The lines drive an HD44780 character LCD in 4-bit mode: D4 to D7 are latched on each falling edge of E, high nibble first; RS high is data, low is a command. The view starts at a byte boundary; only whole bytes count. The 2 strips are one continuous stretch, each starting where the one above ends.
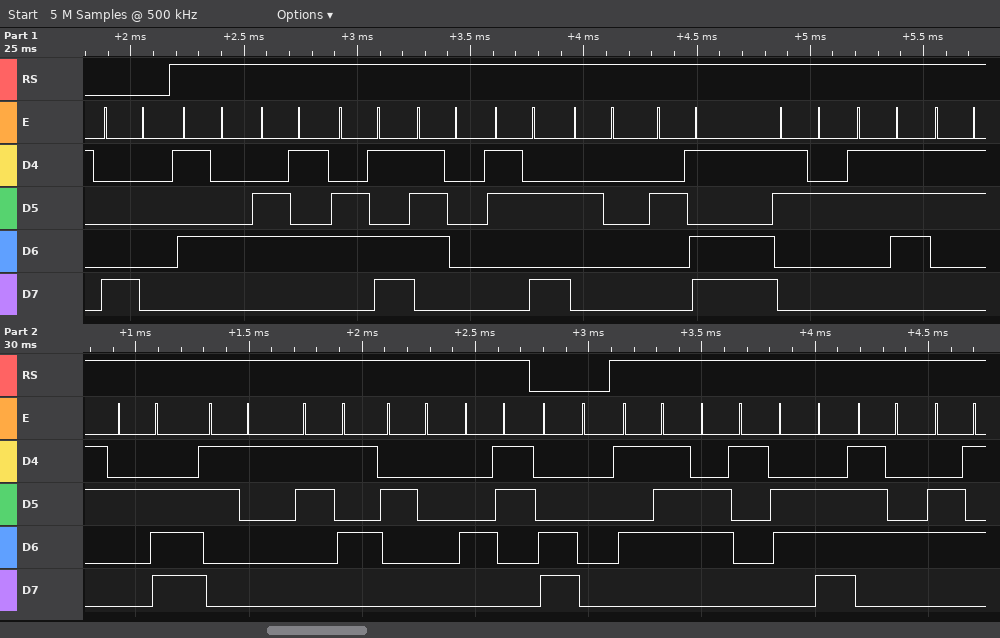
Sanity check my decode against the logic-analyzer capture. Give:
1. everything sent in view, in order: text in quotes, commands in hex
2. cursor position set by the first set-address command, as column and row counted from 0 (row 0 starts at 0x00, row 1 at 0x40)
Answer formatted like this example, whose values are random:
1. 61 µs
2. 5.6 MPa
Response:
1. 0x80 "Temp: -273.15 C" 0xC0 "Wante"
2. column 0, row 0
